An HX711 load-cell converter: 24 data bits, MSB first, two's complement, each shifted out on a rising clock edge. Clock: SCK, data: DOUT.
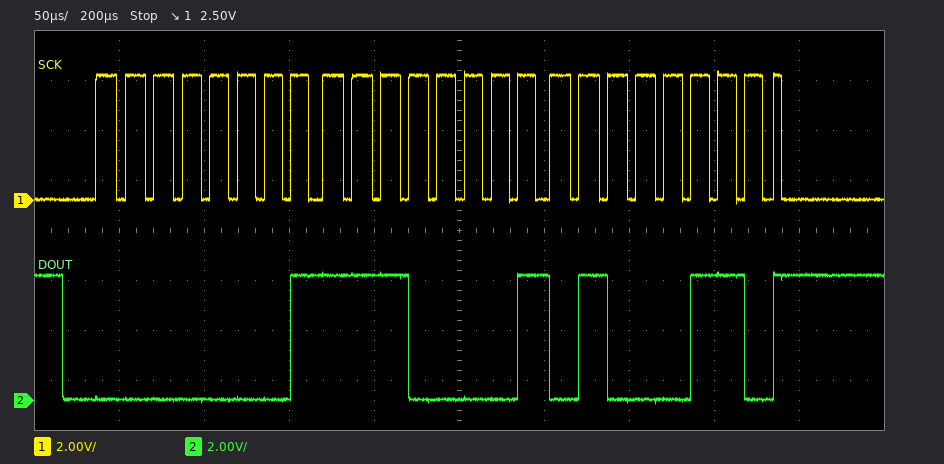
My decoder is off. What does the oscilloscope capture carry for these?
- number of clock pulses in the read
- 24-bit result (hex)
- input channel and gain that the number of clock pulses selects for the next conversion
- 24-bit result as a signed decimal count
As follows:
25
0x01E146
channel A, gain 128
123206
